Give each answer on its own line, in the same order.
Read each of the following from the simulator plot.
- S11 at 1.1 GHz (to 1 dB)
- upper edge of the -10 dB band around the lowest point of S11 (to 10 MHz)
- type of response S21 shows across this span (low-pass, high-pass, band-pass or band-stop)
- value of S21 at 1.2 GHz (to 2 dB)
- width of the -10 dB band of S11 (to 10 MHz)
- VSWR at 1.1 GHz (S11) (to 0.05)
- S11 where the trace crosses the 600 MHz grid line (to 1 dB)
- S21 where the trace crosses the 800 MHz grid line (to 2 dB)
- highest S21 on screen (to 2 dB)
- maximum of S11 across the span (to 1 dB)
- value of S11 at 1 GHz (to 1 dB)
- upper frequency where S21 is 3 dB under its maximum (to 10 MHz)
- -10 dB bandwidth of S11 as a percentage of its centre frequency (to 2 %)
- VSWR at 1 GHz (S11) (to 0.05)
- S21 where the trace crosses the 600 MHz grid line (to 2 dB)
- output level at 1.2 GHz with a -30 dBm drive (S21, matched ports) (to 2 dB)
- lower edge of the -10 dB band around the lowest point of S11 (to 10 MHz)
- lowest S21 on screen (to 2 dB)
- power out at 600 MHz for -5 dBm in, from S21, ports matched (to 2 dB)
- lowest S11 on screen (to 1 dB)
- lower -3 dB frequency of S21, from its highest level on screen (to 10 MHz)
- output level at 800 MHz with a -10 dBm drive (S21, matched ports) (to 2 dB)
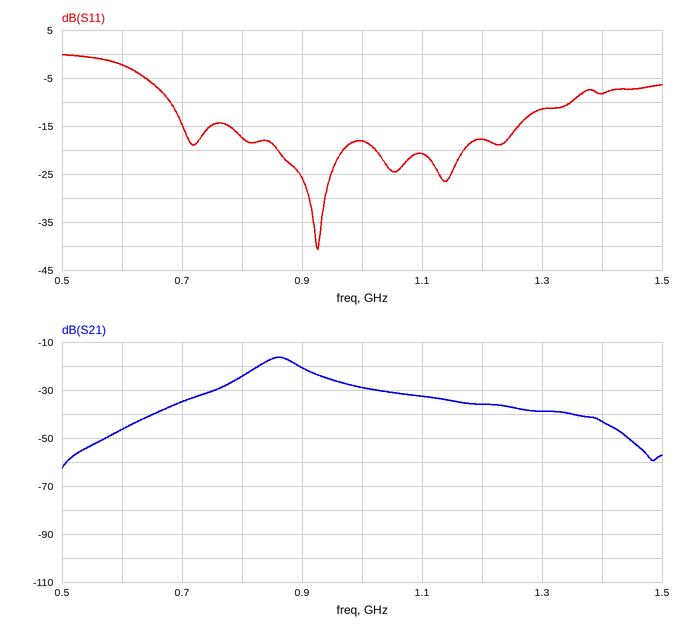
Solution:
-21 dB
1.35 GHz
band-pass
-36 dB
670 MHz
1.20
-2 dB
-24 dB
-16 dB
0 dB
-18 dB
890 MHz
66 %
1.30
-46 dB
-66 dBm
680 MHz
-62 dB
-52 dBm
-41 dB
830 MHz
-34 dBm
